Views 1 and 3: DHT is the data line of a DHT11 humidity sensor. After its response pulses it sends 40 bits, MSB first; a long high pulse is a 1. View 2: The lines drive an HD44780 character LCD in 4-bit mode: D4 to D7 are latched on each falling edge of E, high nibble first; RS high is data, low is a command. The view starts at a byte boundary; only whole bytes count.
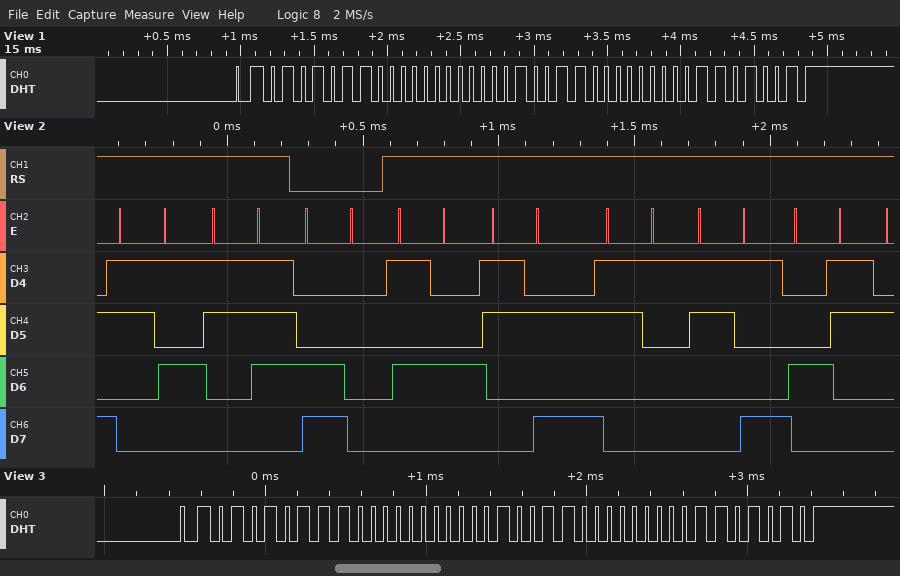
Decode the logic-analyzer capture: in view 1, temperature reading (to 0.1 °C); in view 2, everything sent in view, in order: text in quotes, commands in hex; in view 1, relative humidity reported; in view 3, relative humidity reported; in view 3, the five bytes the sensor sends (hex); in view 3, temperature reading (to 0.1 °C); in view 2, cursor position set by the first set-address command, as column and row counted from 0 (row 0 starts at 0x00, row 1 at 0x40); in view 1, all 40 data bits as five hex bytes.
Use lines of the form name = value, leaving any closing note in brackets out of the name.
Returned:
in view 1, temperature reading = 19.0 °C
in view 2, everything sent in view, in order: text in quotes, commands in hex = "57" 0xC0 "T:19C"
in view 1, relative humidity reported = 86 %
in view 3, relative humidity reported = 87 %
in view 3, the five bytes the sensor sends = 57 00 13 00 6A
in view 3, temperature reading = 19.0 °C
in view 2, cursor position set by the first set-address command, as column and row counted from 0 = column 0, row 1
in view 1, all 40 data bits as five hex bytes = 56 00 13 00 69
